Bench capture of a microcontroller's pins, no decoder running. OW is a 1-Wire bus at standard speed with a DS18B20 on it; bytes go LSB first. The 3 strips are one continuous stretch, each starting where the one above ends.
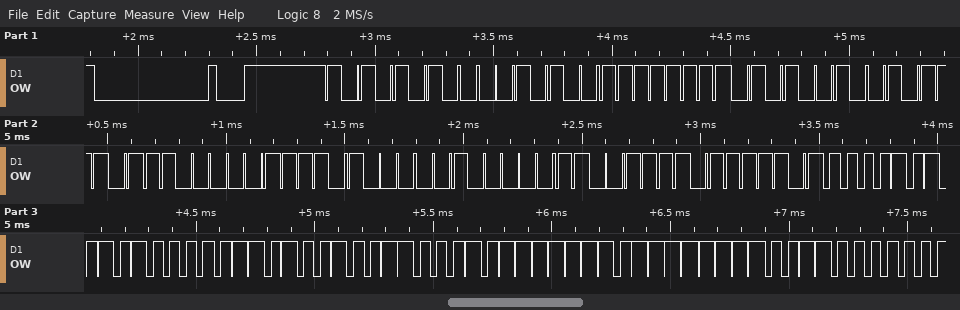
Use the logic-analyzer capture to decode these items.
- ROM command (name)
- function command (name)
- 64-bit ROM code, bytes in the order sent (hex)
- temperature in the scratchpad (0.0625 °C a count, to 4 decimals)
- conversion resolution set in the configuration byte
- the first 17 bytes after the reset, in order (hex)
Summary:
Match ROM
Read Scratchpad
28 FF 4A BA 83 17 04 F3
85.0000 °C
12 bits
55 28 FF 4A BA 83 17 04 F3 BE 50 05 4B 46 7F FF 0C
